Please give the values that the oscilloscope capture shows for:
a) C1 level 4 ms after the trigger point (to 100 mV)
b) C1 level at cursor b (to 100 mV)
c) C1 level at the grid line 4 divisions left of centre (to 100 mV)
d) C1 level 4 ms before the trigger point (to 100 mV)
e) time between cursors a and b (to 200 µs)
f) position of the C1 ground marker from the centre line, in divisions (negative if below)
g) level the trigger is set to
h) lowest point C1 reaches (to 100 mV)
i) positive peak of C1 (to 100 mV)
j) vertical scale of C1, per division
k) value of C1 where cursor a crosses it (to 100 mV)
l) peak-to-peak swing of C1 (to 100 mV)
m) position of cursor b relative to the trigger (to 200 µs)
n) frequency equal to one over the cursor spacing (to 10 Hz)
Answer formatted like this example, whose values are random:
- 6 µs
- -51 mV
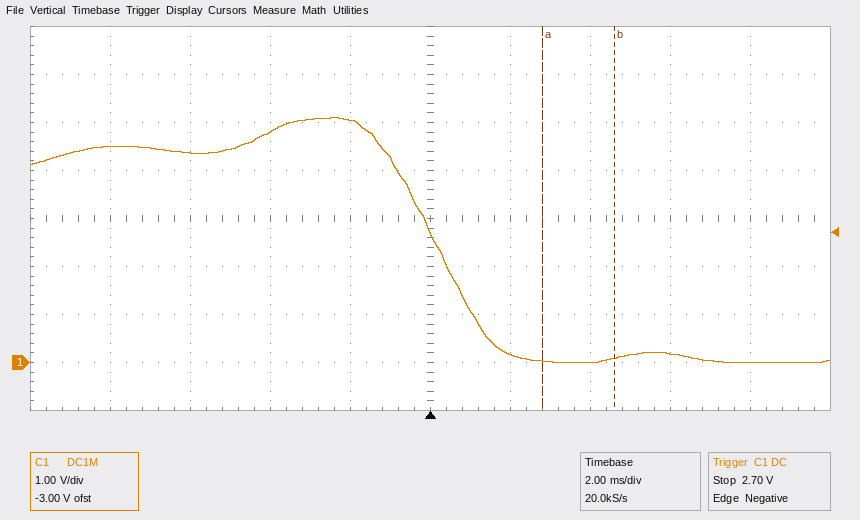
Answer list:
- 0.0 V
- 100 mV
- 4.5 V
- 4.8 V
- 1.8 ms
- -3.0 div
- 2.70 V
- 0.0 V
- 5.1 V
- 1 V
- 0.0 V
- 5.1 V
- +4.6 ms
- 560 Hz
